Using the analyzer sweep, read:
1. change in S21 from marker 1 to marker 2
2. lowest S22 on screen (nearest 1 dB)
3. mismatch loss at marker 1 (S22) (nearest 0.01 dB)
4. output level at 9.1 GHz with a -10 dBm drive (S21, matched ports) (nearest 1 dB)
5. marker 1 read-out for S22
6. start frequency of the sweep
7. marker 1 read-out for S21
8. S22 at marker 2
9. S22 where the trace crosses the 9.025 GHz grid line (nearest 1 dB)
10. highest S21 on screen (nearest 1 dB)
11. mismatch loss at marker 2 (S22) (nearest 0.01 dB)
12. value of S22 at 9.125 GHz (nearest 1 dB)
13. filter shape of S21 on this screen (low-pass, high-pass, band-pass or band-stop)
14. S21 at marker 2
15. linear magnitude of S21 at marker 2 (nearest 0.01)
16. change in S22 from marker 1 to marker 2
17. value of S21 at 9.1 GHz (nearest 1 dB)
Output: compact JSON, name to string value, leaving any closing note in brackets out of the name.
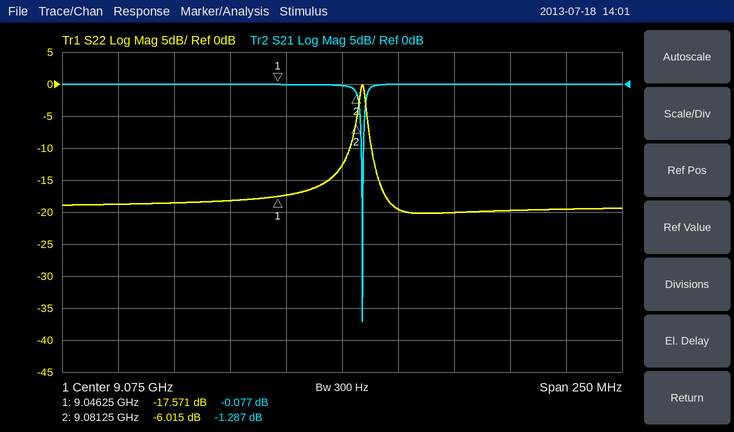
{"change in S21 from marker 1 to marker 2": "-1.210 dB", "lowest S22 on screen": "-20 dB", "mismatch loss at marker 1 (S22)": "0.08 dB", "output level at 9.1 GHz with a -10 dBm drive (S21, matched ports)": "-10 dBm", "marker 1 read-out for S22": "-17.571 dB", "start frequency of the sweep": "8.95 GHz", "marker 1 read-out for S21": "-0.077 dB", "S22 at marker 2": "-6.015 dB", "S22 where the trace crosses the 9.025 GHz grid line": "-18 dB", "highest S21 on screen": "0 dB", "mismatch loss at marker 2 (S22)": "1.25 dB", "value of S22 at 9.125 GHz": "-20 dB", "filter shape of S21 on this screen": "band-stop", "S21 at marker 2": "-1.287 dB", "linear magnitude of S21 at marker 2": "0.86", "change in S22 from marker 1 to marker 2": "11.556 dB", "value of S21 at 9.1 GHz": "0 dB"}
